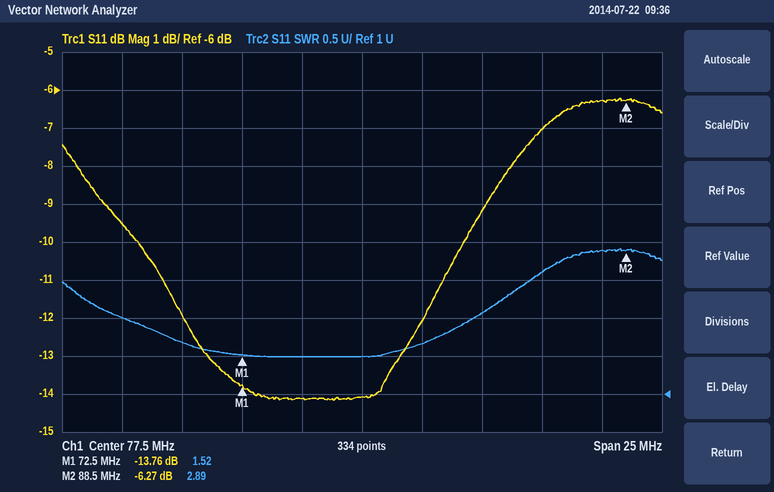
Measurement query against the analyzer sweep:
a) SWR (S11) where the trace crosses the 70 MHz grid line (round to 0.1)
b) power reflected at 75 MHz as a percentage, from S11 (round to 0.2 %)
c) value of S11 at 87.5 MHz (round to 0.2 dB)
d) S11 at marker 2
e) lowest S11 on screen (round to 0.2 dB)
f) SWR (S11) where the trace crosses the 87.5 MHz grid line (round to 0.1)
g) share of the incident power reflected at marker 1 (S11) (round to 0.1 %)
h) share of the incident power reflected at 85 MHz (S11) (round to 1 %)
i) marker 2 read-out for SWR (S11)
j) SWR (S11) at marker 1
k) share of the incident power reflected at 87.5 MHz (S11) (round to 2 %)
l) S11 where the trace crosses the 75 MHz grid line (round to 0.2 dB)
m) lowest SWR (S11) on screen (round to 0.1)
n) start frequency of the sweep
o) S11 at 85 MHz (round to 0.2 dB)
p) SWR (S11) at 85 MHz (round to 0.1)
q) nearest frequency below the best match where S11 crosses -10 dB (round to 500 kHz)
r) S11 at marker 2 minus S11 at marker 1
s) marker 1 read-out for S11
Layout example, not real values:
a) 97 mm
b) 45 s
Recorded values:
a) 1.7
b) 3.8 %
c) -6.2 dB
d) -6.27 dB
e) -14.2 dB
f) 2.9
g) 4.2 %
h) 20 %
i) 2.89
j) 1.52
k) 24 %
l) -14.2 dB
m) 1.5
n) 65 MHz
o) -7.0 dB
p) 2.6
q) 68.0 MHz
r) 7.49 dB
s) -13.76 dB
